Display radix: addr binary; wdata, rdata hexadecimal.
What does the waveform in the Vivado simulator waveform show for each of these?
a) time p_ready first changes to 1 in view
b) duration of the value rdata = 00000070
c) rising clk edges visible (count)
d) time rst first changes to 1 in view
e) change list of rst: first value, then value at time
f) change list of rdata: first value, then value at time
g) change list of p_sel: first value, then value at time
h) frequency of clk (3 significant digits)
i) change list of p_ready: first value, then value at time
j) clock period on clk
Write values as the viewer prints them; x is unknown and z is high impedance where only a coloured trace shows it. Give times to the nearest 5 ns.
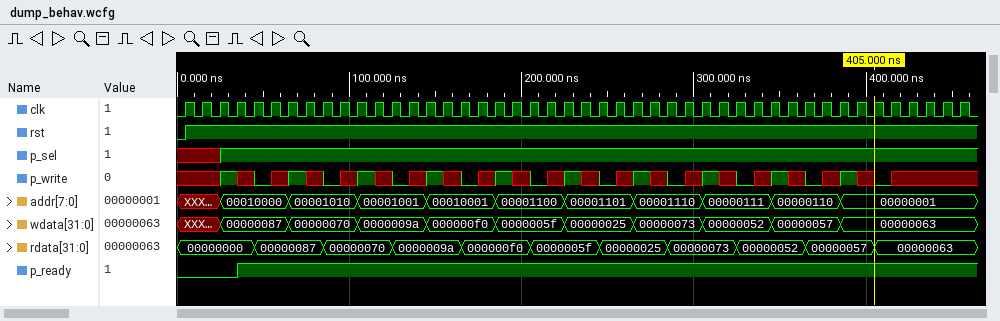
35 ns
40 ns
46
5 ns
0, 1 at 5 ns
00000000, 00000087 at 45 ns, 00000070 at 85 ns, 0000009a at 125 ns, 000000f0 at 165 ns, 0000005f at 205 ns, 00000025 at 245 ns, 00000073 at 285 ns, 00000052 at 325 ns, 00000057 at 365 ns, 00000063 at 405 ns
x, 1 at 25 ns
100 MHz
0, 1 at 35 ns
10 ns
